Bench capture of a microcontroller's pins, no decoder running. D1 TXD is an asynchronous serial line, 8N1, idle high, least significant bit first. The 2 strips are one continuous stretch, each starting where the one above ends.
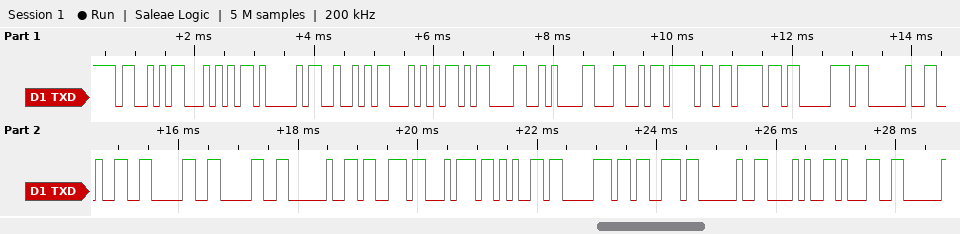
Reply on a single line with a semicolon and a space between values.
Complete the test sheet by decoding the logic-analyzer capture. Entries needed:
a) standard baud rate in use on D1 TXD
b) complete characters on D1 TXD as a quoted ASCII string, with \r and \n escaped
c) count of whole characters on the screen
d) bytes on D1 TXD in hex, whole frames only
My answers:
9600 baud; "START\r\nLoop 200 steps (1"; 24; 53 54 41 52 54 0D 0A 4C 6F 6F 70 20 32 30 30 20 73 74 65 70 73 20 28 31
